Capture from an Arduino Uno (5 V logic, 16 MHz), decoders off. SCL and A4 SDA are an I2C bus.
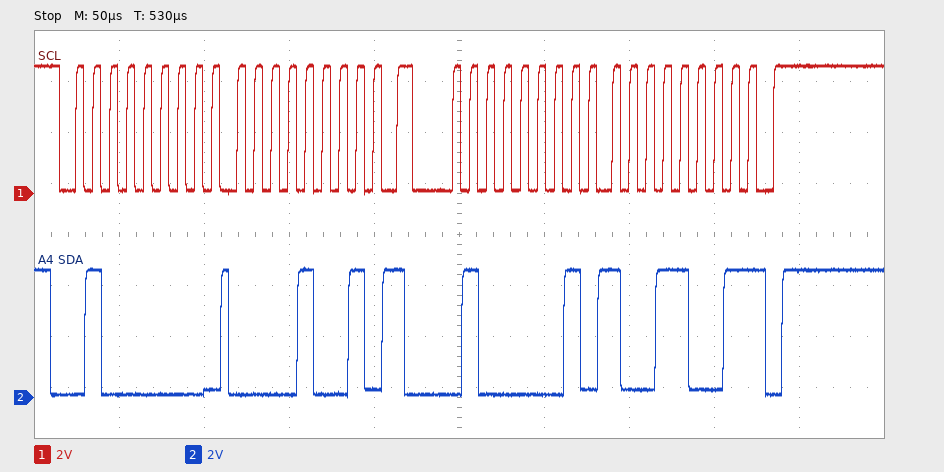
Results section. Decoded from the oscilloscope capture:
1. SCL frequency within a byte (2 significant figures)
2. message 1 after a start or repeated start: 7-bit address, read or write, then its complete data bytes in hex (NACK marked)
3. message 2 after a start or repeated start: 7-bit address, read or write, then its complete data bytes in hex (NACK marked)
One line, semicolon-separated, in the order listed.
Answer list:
100 kHz; 0x20 write: 09; 0x20 read: 99 NACK
